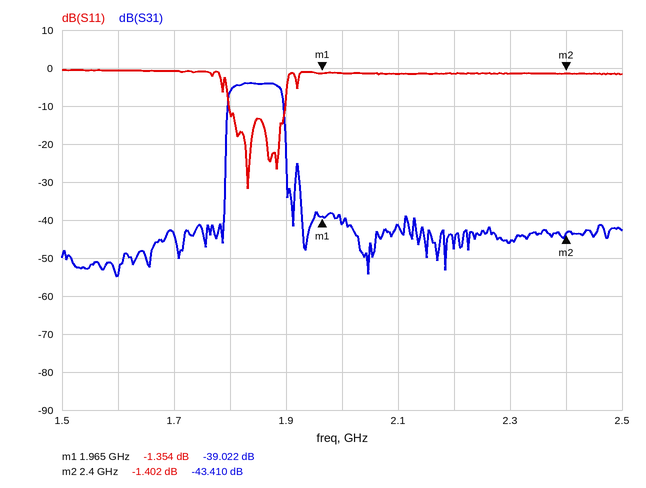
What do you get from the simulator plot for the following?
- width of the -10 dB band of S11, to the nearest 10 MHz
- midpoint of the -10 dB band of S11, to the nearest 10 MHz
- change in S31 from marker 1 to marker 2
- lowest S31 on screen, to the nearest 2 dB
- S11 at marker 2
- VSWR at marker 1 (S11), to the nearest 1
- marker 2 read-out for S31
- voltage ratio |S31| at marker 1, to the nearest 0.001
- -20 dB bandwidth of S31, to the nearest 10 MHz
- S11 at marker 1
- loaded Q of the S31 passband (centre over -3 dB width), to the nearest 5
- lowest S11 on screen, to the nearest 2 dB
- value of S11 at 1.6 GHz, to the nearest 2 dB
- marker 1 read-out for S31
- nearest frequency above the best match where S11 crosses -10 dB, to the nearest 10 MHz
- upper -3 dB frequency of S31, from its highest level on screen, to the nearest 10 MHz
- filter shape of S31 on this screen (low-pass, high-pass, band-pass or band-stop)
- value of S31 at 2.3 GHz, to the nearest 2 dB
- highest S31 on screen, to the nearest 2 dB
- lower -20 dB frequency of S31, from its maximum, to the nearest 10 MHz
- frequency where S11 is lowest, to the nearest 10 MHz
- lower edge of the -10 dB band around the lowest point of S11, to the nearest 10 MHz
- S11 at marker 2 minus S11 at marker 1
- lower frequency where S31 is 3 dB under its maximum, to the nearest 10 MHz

100 MHz
1.85 GHz
-4.388 dB
-54 dB
-1.402 dB
13
-43.410 dB
0.011
110 MHz
-1.354 dB
20
-32 dB
0 dB
-39.022 dB
1.90 GHz
1.89 GHz
band-pass
-46 dB
-4 dB
1.79 GHz
1.83 GHz
1.80 GHz
-0.048 dB
1.80 GHz
